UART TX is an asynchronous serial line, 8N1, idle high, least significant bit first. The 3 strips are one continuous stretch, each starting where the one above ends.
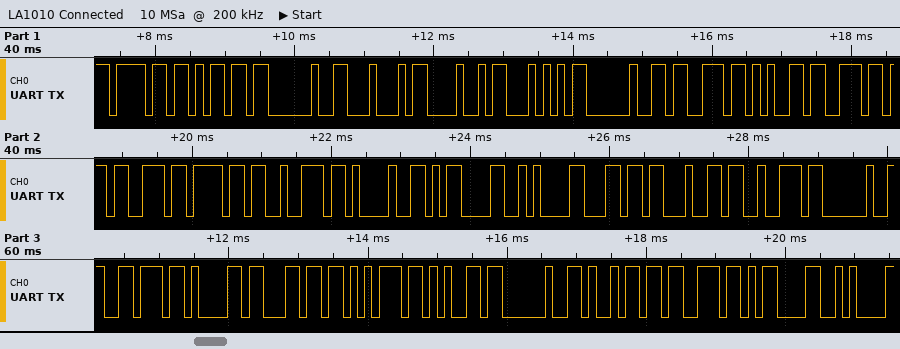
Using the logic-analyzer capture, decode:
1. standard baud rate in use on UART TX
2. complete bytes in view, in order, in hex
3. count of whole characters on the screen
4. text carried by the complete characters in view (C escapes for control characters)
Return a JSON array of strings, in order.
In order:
["9600 baud", "6F 6D 20 44 48 54 20 73 65 6E 73 6F 72 21 0D 0A 6C 64 72 20 76 61 6C 75 65 20 69 73 0D 0A", "30", "\"om DHT sensor!\\r\\nldr value is\\r\\n\""]
